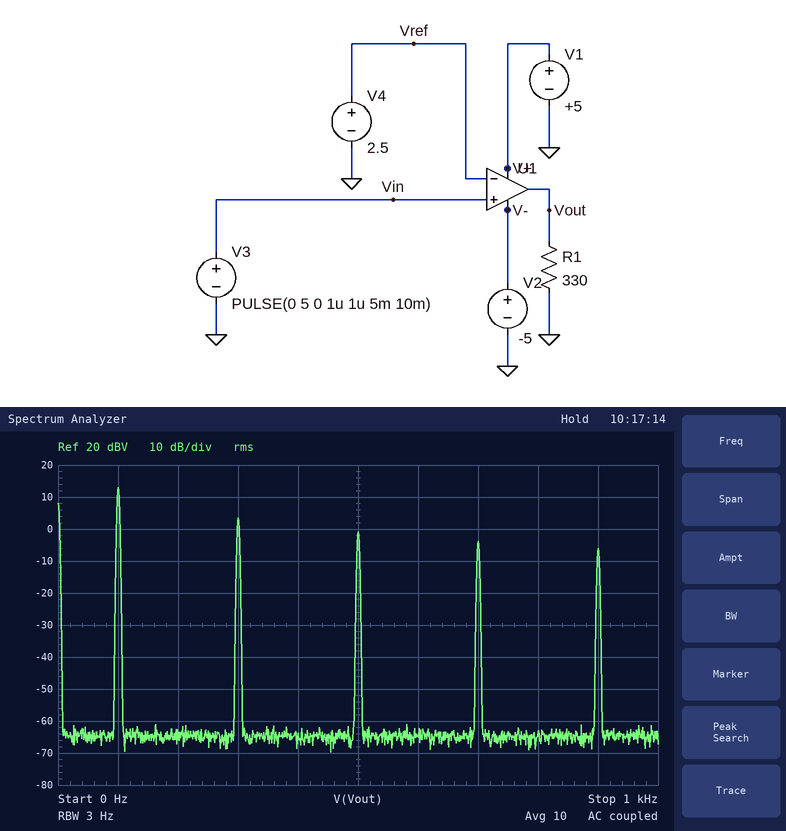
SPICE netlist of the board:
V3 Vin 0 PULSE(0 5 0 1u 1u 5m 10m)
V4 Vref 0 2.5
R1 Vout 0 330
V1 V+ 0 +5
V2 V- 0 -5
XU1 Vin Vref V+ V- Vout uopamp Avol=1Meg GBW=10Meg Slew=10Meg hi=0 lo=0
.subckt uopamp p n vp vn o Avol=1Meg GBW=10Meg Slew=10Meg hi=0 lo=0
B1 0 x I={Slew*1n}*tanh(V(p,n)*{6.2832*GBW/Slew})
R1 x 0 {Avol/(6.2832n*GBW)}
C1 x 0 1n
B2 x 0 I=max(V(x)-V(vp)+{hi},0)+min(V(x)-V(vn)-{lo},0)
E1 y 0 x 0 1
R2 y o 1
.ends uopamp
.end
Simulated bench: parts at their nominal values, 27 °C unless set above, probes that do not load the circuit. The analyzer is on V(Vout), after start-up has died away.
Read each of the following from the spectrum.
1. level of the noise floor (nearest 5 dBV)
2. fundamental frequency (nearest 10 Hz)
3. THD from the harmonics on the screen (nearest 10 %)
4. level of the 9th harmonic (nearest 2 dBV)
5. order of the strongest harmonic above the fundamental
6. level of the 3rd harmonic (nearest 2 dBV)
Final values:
-65 dBV
100 Hz
40 %
-6 dBV
3
4 dBV
